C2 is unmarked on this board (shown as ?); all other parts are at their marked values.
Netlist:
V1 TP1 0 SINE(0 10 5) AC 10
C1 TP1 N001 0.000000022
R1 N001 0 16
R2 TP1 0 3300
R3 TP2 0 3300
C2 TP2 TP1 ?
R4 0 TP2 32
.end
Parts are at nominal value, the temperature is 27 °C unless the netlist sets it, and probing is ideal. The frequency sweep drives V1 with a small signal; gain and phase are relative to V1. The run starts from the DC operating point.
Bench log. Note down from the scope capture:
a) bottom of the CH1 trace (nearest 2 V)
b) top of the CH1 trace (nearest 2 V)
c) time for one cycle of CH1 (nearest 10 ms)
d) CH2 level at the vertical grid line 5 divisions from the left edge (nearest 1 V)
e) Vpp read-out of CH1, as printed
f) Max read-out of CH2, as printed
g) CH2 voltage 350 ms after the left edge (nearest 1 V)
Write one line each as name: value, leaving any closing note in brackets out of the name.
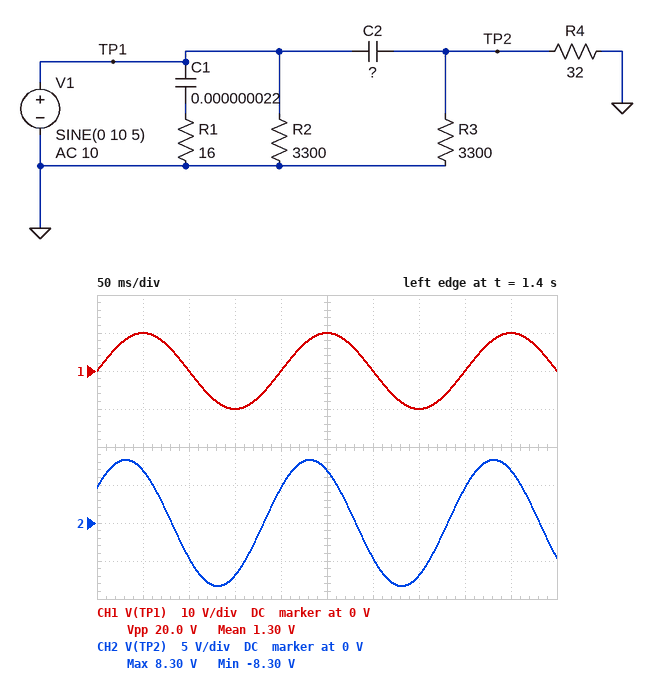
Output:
bottom of the CH1 trace: -10 V
top of the CH1 trace: 10 V
time for one cycle of CH1: 200 ms
CH2 level at the vertical grid line 5 divisions from the left edge: 7 V
Vpp read-out of CH1, as printed: 20.0 V
Max read-out of CH2, as printed: 8.30 V
CH2 voltage 350 ms after the left edge: -7 V
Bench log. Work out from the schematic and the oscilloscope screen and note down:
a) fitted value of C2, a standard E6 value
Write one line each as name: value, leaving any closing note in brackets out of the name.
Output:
fitted value of C2, a standard E6 value: 1.5 mF
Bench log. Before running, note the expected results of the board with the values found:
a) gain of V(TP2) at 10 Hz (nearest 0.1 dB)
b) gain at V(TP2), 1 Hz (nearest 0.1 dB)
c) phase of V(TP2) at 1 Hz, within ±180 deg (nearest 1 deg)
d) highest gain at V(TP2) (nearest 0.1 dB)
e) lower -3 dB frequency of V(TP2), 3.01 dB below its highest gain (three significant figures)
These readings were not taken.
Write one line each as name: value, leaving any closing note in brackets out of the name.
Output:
gain of V(TP2) at 10 Hz: -0.5 dB
gain at V(TP2), 1 Hz: -10.9 dB
phase of V(TP2) at 1 Hz, within ±180 deg: 73 deg
highest gain at V(TP2): 0 dB
lower -3 dB frequency of V(TP2), 3.01 dB below its highest gain: 3.35 Hz
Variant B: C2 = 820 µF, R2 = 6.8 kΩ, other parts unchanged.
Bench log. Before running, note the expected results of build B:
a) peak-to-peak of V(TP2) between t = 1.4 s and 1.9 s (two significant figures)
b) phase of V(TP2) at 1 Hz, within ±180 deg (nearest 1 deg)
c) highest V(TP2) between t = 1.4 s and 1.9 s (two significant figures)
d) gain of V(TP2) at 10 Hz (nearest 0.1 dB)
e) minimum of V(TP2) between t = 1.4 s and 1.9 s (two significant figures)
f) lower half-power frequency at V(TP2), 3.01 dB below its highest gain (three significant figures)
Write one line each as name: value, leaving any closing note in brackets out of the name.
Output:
peak-to-peak of V(TP2) between t = 1.4 s and 1.9 s: 13 V
phase of V(TP2) at 1 Hz, within ±180 deg: 81 deg
highest V(TP2) between t = 1.4 s and 1.9 s: 6.3 V
gain of V(TP2) at 10 Hz: -1.4 dB
minimum of V(TP2) between t = 1.4 s and 1.9 s: -6.3 V
lower half-power frequency at V(TP2), 3.01 dB below its highest gain: 6.12 Hz
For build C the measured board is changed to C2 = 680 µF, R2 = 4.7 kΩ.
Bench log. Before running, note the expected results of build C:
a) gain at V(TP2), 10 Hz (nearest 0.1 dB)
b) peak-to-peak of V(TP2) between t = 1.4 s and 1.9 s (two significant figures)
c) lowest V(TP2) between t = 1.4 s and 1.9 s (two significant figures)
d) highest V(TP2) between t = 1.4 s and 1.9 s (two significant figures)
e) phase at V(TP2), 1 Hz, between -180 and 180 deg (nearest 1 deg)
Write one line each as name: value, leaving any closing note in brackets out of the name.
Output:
gain at V(TP2), 10 Hz: -1.9 dB
peak-to-peak of V(TP2) between t = 1.4 s and 1.9 s: 11 V
lowest V(TP2) between t = 1.4 s and 1.9 s: -5.6 V
highest V(TP2) between t = 1.4 s and 1.9 s: 5.6 V
phase at V(TP2), 1 Hz, between -180 and 180 deg: 82 deg
